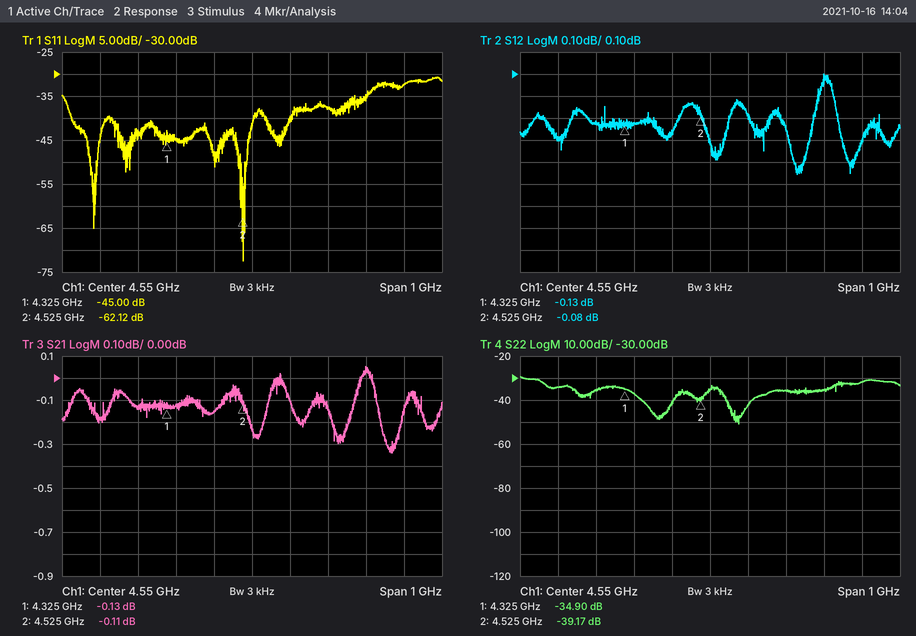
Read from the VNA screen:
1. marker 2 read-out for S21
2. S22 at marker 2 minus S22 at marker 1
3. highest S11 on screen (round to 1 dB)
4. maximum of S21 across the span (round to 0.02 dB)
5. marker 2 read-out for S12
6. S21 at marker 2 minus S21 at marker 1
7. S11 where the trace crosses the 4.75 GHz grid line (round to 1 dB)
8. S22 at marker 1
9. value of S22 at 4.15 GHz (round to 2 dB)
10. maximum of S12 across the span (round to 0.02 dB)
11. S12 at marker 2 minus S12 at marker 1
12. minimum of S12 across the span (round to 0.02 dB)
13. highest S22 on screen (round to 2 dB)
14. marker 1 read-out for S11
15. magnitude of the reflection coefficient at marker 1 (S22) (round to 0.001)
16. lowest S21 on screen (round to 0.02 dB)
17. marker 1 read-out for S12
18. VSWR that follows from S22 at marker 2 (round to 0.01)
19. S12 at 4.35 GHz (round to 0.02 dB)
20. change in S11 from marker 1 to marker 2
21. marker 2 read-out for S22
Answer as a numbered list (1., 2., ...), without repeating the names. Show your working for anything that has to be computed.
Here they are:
1. -0.11 dB
2. -39.17 − (-34.9) = -4.27 dB
3. -31 dB
4. 0.06 dB
5. -0.08 dB
6. -0.11 − (-0.13) = 0.02 dB
7. -38 dB
8. -34.90 dB
9. -34 dB
10. 0.10 dB
11. -0.08 − (-0.13) = 0.05 dB
12. -0.36 dB
13. -30 dB
14. -45.00 dB
15. 10^(-34.9/20) ≈ 0.018
16. -0.34 dB
17. -0.13 dB
18. (1 + 0.0110)/(1 − 0.0110) ≈ 1.02
19. -0.12 dB
20. -62.12 − (-45) = -17.12 dB
21. -39.17 dB
